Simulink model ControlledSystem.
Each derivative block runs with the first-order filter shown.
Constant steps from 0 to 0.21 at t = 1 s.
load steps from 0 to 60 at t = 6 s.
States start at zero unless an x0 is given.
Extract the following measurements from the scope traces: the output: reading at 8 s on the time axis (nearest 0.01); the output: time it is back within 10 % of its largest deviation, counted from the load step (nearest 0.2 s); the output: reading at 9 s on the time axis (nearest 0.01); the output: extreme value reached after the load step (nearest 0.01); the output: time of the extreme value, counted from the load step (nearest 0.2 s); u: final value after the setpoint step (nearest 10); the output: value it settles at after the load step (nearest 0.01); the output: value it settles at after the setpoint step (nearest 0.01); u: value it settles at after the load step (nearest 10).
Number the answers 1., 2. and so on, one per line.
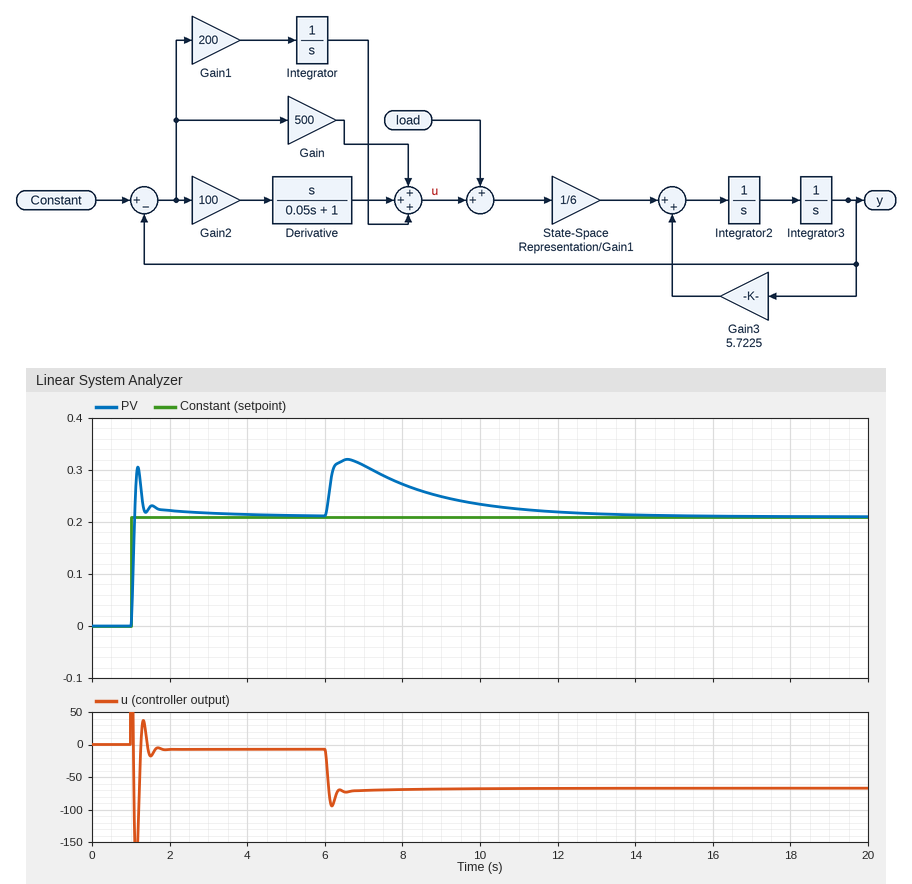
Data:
1. 0.27
2. 5.6 s
3. 0.25
4. 0.32
5. 0.6 s
6. -10
7. 0.21
8. 0.21
9. -70
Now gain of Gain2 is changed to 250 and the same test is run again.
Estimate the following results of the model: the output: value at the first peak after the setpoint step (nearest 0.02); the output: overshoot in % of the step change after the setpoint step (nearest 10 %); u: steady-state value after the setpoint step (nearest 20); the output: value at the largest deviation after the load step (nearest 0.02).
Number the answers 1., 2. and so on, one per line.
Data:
1. 0.30
2. 40 %
3. 0
4. 0.30
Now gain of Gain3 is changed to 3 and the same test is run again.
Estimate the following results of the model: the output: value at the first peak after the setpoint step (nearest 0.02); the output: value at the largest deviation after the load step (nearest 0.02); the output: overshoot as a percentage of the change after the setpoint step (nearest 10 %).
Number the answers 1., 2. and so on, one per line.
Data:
1. 0.30
2. 0.32
3. 40 %
